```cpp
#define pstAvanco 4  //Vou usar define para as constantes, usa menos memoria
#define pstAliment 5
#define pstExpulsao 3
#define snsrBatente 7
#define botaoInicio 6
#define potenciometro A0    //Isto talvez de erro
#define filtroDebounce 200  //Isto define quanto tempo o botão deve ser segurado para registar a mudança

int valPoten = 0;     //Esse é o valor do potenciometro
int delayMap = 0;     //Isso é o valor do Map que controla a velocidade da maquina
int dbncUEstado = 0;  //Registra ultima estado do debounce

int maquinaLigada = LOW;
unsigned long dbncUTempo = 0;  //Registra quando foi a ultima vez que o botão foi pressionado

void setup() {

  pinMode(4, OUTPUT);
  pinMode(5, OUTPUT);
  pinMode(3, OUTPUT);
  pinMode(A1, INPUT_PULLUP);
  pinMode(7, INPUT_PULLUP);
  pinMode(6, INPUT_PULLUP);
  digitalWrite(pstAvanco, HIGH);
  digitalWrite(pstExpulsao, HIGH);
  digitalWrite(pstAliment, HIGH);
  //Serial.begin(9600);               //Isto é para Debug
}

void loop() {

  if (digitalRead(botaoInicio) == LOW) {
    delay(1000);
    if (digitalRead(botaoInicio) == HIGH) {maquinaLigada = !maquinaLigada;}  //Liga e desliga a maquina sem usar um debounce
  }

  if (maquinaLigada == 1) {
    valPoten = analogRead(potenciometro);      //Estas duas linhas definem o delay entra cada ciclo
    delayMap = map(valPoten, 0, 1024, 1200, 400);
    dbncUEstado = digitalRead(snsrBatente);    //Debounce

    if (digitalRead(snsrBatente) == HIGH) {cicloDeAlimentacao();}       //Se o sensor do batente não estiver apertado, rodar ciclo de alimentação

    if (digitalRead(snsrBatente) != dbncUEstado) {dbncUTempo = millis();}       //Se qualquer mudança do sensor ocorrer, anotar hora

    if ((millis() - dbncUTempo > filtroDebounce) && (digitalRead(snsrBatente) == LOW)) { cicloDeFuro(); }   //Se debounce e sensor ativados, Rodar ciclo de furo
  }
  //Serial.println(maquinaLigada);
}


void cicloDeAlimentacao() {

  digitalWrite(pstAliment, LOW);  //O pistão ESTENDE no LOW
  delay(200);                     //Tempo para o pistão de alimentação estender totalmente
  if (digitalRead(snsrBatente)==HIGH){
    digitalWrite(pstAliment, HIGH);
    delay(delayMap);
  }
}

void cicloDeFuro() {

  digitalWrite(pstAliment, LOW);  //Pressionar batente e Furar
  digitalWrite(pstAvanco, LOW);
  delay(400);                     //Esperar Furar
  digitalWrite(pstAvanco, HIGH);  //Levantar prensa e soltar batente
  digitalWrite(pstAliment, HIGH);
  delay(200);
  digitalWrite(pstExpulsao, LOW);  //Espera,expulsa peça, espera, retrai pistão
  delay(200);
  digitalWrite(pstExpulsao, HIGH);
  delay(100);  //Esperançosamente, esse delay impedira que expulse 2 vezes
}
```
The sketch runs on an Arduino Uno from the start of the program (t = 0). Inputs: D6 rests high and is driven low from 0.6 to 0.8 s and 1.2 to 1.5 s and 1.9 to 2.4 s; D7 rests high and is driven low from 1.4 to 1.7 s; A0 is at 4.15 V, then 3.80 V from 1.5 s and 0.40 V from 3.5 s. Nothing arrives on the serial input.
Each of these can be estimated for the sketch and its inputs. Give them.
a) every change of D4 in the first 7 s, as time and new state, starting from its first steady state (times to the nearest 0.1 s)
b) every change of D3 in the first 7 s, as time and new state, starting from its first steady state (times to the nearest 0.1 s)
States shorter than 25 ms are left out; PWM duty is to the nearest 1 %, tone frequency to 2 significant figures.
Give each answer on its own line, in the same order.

0 s high; 1.6 s low; 2 s high
0 s high; 2.2 s low; 2.4 s high
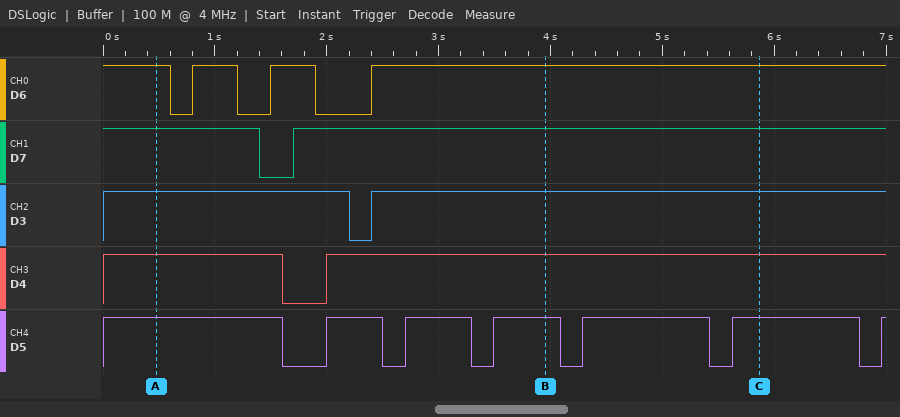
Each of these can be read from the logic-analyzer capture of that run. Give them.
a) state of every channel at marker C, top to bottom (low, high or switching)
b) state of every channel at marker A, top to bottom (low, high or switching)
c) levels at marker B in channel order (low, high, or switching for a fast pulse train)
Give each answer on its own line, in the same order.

D6 high, D7 high, D3 high, D4 high, D5 high
D6 high, D7 high, D3 high, D4 high, D5 high
D6 high, D7 high, D3 high, D4 high, D5 high
